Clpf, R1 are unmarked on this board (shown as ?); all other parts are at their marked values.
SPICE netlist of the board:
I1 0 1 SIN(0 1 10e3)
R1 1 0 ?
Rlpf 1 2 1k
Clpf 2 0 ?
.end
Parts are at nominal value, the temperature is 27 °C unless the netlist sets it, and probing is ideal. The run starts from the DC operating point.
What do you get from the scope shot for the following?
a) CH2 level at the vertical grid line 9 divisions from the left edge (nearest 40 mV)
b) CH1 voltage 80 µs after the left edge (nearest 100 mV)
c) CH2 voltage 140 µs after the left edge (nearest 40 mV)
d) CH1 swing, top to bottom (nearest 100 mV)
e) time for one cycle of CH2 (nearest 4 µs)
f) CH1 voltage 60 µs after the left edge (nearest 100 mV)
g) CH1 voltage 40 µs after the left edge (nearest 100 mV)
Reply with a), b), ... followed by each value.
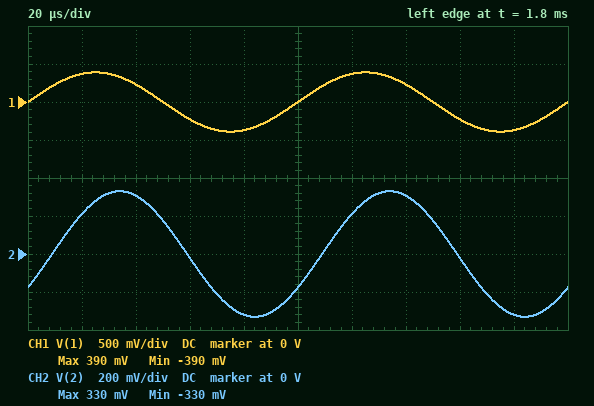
a) -320 mV
b) -400 mV
c) 320 mV
d) 800 mV
e) 100 µs
f) -200 mV
g) 200 mV
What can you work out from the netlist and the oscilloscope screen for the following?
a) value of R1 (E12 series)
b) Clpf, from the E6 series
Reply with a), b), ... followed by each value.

a) 0.39 Ω
b) 10 nF
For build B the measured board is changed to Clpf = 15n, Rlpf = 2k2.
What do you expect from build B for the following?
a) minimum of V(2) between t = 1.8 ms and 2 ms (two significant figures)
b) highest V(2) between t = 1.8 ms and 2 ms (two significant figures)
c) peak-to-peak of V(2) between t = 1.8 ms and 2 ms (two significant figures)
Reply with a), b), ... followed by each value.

a) -170 mV
b) 170 mV
c) 340 mV
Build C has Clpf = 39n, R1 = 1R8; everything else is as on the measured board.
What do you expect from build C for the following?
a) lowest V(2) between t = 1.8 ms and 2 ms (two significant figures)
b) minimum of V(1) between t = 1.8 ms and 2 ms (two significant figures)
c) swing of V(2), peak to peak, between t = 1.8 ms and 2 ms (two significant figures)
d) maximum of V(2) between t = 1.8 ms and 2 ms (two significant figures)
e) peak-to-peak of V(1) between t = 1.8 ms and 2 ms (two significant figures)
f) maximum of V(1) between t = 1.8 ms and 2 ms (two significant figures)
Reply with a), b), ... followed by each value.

a) -680 mV
b) -1.8 V
c) 1.4 V
d) 680 mV
e) 3.6 V
f) 1.8 V
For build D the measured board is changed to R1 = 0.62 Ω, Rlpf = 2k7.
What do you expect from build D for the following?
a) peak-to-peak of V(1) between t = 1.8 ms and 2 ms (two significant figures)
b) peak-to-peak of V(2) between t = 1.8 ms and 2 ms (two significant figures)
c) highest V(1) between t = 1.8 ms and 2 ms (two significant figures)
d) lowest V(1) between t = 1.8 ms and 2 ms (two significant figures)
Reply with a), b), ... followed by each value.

a) 1.2 V
b) 630 mV
c) 620 mV
d) -620 mV
